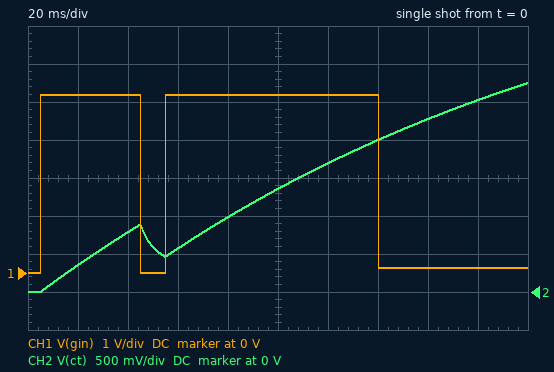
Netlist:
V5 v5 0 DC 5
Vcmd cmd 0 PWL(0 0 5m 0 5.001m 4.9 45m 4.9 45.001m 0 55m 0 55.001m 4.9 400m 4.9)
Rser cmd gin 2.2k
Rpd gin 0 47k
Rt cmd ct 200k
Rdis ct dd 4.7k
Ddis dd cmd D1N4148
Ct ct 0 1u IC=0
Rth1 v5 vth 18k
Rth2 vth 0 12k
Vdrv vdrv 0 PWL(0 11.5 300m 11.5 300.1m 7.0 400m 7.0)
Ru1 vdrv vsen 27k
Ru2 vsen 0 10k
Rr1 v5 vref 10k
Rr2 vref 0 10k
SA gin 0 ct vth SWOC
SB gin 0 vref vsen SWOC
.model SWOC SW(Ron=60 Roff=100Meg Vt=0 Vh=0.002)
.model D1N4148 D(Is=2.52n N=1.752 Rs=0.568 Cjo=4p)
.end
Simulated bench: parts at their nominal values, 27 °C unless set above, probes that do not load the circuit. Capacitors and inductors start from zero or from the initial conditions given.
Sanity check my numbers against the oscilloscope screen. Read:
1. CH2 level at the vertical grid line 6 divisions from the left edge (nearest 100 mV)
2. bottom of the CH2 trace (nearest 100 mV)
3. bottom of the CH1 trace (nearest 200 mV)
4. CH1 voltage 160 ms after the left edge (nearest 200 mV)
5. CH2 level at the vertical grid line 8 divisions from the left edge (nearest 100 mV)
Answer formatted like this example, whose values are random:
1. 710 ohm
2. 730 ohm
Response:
1. 1.7 V
2. 0 V
3. 0 V
4. 200 mV
5. 2.3 V
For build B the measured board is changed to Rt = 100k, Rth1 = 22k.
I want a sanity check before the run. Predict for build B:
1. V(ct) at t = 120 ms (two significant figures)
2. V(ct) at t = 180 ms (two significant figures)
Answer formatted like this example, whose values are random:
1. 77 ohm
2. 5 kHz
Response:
1. 2.6 V
2. 3.7 V
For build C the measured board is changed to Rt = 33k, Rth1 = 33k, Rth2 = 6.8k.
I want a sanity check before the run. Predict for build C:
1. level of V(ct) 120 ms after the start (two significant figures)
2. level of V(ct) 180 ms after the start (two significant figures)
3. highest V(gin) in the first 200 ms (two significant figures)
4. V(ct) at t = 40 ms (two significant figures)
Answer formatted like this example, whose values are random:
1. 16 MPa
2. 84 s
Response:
1. 4.3 V
2. 4.8 V
3. 4.7 V
4. 3.2 V
